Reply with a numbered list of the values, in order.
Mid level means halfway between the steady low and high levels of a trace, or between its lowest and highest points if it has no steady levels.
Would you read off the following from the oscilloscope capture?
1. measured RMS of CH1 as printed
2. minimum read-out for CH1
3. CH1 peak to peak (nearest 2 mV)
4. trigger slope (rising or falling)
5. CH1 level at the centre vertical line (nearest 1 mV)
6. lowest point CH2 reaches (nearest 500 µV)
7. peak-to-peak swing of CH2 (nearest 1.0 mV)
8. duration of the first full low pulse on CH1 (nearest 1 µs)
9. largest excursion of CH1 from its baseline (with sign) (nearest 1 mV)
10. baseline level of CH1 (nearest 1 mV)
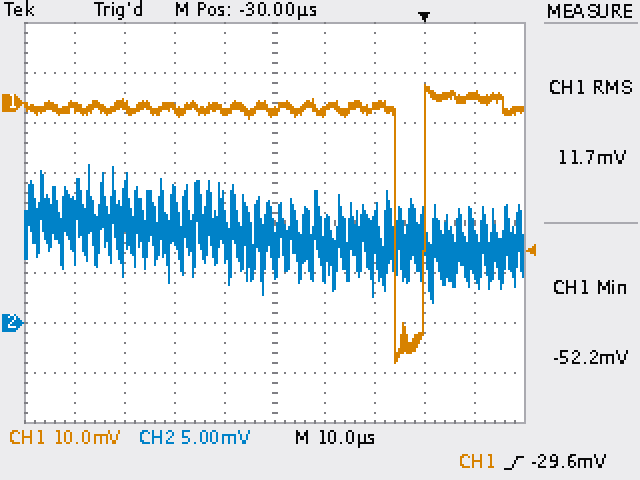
1. 11.7 mV
2. -52.2 mV
3. 56 mV
4. rising
5. -2 mV
6. 2.0 mV
7. 14.0 mV
8. 6 µs
9. -51 mV
10. -1 mV
